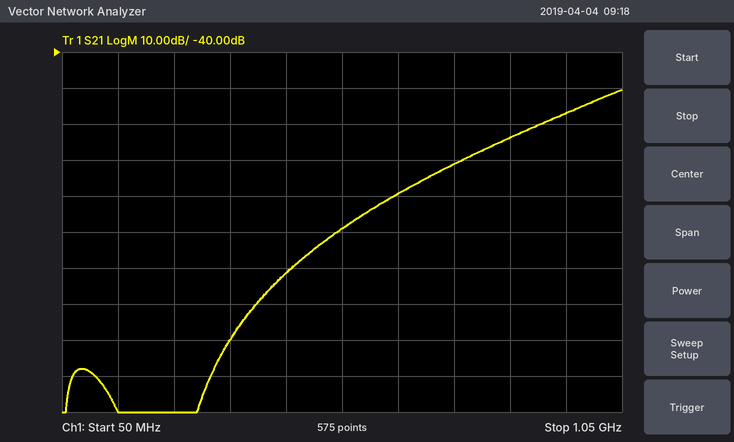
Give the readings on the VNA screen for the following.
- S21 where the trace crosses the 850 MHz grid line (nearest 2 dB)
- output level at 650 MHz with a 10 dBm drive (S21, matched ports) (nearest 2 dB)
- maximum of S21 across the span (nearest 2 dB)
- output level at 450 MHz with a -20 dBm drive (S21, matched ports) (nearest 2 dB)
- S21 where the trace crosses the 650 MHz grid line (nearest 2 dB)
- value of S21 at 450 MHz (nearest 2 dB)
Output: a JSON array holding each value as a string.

["-64 dB", "-70 dBm", "-50 dB", "-122 dBm", "-80 dB", "-102 dB"]
